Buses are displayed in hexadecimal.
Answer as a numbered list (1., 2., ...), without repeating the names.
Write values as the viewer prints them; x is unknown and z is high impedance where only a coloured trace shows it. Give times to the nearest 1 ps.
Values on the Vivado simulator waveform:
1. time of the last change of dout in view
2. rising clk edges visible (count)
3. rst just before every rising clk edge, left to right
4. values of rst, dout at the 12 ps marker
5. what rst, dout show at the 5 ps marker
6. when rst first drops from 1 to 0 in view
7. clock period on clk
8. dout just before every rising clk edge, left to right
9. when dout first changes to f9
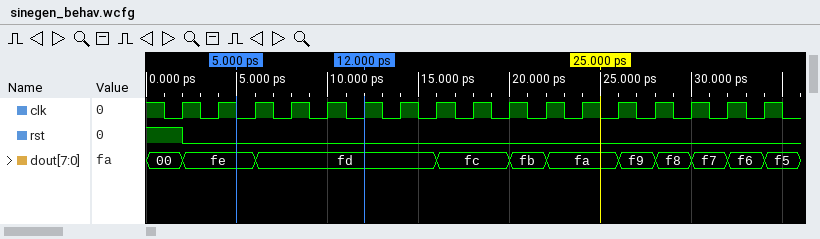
1. 34 ps
2. 17
3. 1 0 0 0 0 0 0 0 0 0 0 0 0 0 0 0 0
4. rst=0, dout=fd
5. rst=0, dout=fe
6. 2 ps
7. 2 ps
8. 00, fe, fe, fd, fd, fd, fd, fd, fc, fc, fb, fa, fa, f9, f8, f7, f6
9. 26 ps
